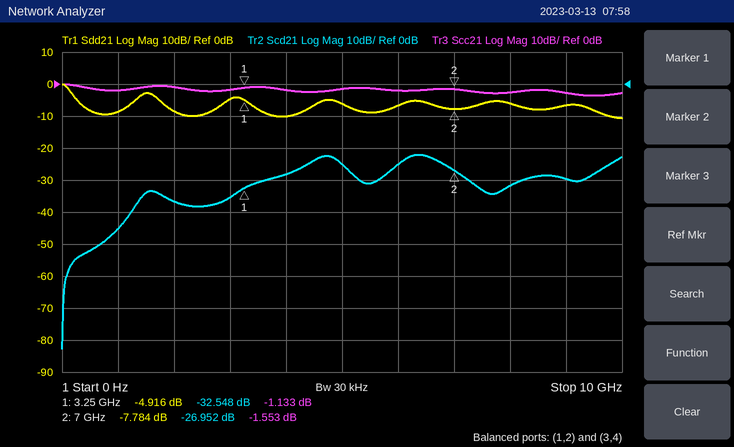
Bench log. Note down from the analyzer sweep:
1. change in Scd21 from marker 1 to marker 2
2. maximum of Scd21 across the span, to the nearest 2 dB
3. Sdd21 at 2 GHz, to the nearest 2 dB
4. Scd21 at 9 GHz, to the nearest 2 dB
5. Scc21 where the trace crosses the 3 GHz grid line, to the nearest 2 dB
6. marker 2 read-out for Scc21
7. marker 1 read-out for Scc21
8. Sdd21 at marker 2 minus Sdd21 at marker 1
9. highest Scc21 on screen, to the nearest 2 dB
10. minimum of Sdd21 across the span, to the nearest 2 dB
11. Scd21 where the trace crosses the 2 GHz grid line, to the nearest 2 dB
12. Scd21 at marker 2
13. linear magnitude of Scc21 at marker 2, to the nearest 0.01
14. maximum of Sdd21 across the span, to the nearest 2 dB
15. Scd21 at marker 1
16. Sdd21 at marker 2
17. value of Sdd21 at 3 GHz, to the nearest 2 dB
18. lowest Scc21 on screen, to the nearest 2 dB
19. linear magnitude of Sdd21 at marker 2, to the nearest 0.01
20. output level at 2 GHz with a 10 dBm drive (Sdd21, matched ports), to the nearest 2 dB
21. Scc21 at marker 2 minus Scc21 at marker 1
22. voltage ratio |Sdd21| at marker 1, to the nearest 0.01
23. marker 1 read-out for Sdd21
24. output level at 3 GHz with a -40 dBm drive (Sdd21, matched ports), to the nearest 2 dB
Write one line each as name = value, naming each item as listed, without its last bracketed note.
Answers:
change in Scd21 from marker 1 to marker 2 = 5.596 dB
maximum of Scd21 across the span, to the nearest 2 dB = -22 dB
Sdd21 at 2 GHz, to the nearest 2 dB = -8 dB
Scd21 at 9 GHz, to the nearest 2 dB = -30 dB
Scc21 where the trace crosses the 3 GHz grid line, to the nearest 2 dB = -2 dB
marker 2 read-out for Scc21 = -1.553 dB
marker 1 read-out for Scc21 = -1.133 dB
Sdd21 at marker 2 minus Sdd21 at marker 1 = -2.868 dB
highest Scc21 on screen, to the nearest 2 dB = 0 dB
minimum of Sdd21 across the span, to the nearest 2 dB = -10 dB
Scd21 where the trace crosses the 2 GHz grid line, to the nearest 2 dB = -36 dB
Scd21 at marker 2 = -26.952 dB
linear magnitude of Scc21 at marker 2, to the nearest 0.01 = 0.84
maximum of Sdd21 across the span, to the nearest 2 dB = 0 dB
Scd21 at marker 1 = -32.548 dB
Sdd21 at marker 2 = -7.784 dB
value of Sdd21 at 3 GHz, to the nearest 2 dB = -4 dB
lowest Scc21 on screen, to the nearest 2 dB = -4 dB
linear magnitude of Sdd21 at marker 2, to the nearest 0.01 = 0.41
output level at 2 GHz with a 10 dBm drive (Sdd21, matched ports), to the nearest 2 dB = 2 dBm
Scc21 at marker 2 minus Scc21 at marker 1 = -0.420 dB
voltage ratio |Sdd21| at marker 1, to the nearest 0.01 = 0.57
marker 1 read-out for Sdd21 = -4.916 dB
output level at 3 GHz with a -40 dBm drive (Sdd21, matched ports), to the nearest 2 dB = -44 dBm
